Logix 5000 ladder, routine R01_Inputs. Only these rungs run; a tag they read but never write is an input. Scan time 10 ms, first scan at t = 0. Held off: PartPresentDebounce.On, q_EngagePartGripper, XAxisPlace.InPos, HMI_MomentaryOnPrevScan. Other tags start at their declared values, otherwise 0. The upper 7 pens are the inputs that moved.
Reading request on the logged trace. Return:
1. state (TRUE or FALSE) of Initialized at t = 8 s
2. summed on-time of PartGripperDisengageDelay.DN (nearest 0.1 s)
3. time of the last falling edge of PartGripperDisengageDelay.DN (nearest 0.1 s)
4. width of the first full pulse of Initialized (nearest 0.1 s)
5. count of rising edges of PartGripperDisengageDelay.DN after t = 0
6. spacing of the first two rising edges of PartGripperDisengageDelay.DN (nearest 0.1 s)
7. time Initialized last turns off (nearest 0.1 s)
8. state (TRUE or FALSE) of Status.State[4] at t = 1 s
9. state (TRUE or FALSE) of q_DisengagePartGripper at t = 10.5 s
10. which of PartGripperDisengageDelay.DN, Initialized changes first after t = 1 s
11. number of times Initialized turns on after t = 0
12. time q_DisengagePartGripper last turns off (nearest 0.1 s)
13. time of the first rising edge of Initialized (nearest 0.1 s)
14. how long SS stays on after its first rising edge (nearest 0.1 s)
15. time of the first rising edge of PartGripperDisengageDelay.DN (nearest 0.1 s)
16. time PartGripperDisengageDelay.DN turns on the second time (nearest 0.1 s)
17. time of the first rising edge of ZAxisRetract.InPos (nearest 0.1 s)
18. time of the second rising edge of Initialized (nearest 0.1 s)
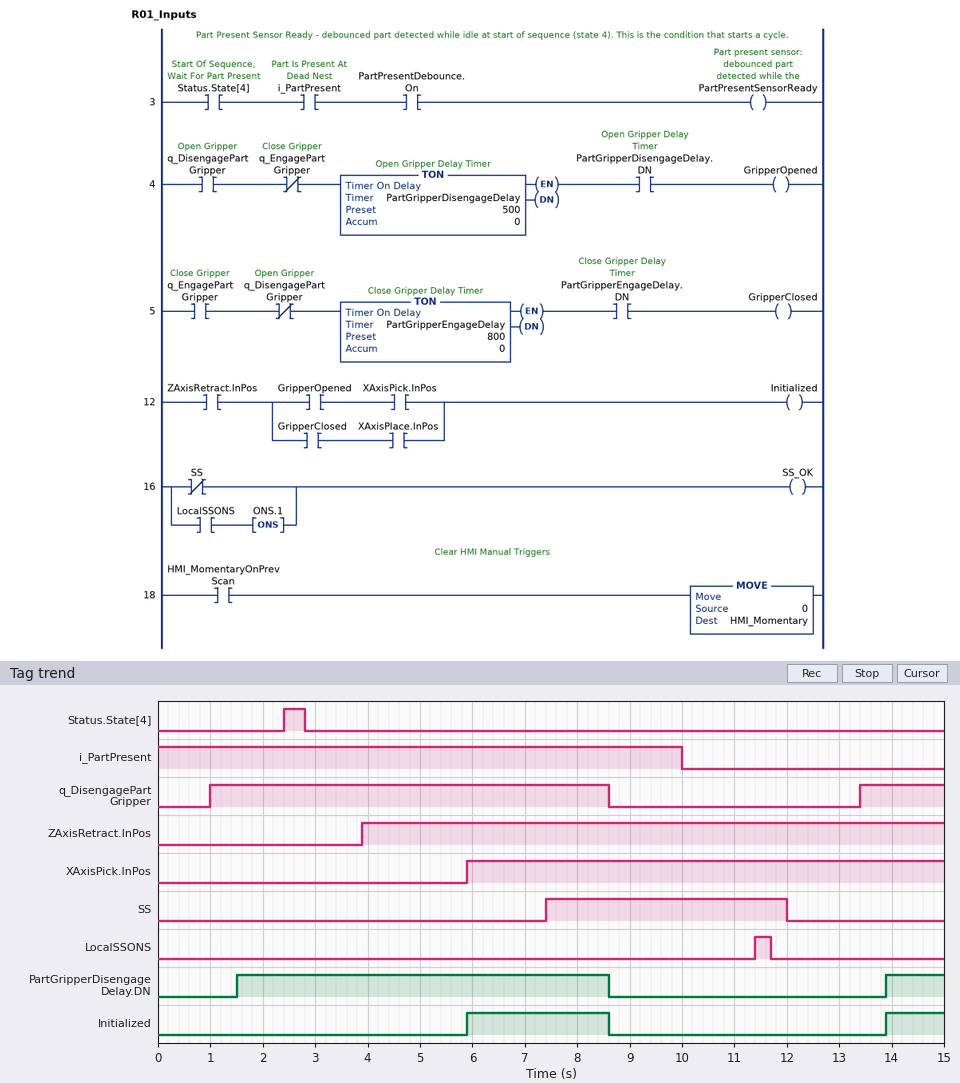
TRUE
8.2 s
8.6 s
2.7 s
2
12.4 s
8.6 s
FALSE
FALSE
PartGripperDisengageDelay.DN
2
8.6 s
5.9 s
4.6 s
1.5 s
13.9 s
3.9 s
13.9 s
